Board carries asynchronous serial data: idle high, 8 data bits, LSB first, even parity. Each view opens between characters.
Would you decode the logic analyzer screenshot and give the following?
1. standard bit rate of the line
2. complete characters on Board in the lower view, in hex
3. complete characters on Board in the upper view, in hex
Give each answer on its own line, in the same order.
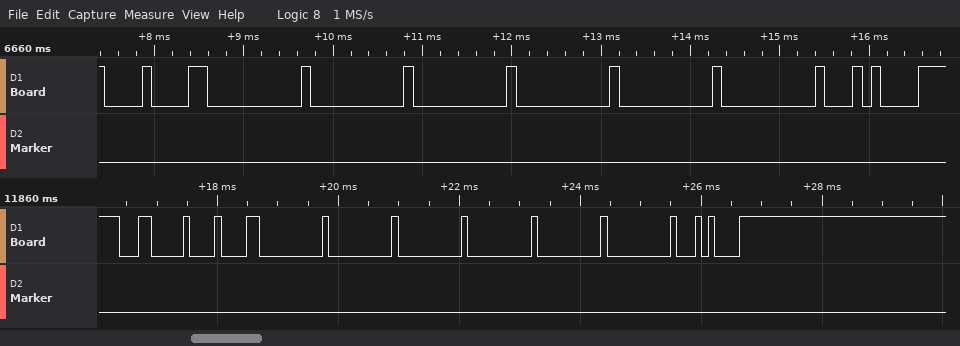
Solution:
9600 baud
0C, 08, 00, 00, 00, 00, 00, 00, 14
08, 00, 00, 00, 00, 00, 00, 14
